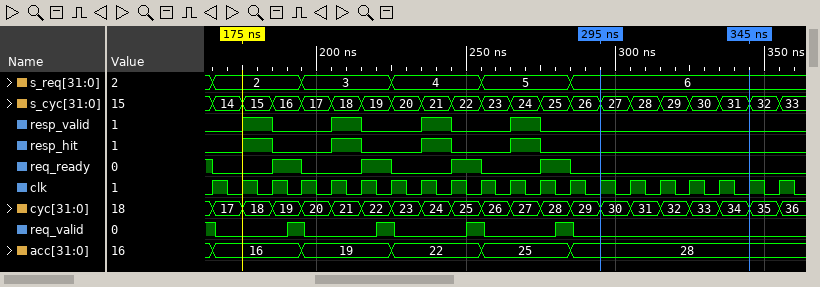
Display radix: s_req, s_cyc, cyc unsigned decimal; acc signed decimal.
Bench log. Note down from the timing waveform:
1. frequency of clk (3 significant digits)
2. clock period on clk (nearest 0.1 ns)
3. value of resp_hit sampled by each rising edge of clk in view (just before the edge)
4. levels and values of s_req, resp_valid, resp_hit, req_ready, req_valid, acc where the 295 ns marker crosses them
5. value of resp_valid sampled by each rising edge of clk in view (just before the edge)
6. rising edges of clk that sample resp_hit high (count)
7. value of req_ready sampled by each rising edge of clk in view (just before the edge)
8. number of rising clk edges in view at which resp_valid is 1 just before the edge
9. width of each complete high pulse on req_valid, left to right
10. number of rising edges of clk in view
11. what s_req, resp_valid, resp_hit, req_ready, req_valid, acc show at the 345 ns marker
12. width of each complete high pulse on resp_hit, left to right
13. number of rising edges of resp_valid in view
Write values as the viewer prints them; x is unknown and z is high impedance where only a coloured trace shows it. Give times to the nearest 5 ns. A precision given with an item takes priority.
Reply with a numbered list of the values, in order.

1. 100 MHz
2. 10 ns
3. 0 0 1 0 0 1 0 0 1 0 0 1 0 0 0 0 0 0 0 0
4. s_req=6, resp_valid=0, resp_hit=0, req_ready=0, req_valid=0, acc=28
5. 0 0 1 0 0 1 0 0 1 0 0 1 0 0 0 0 0 0 0 0
6. 4
7. 1 0 0 1 0 0 1 0 0 1 0 0 1 0 0 0 0 0 0 0
8. 4
9. 5 ns, 5 ns, 5 ns, 5 ns
10. 20
11. s_req=6, resp_valid=0, resp_hit=0, req_ready=0, req_valid=0, acc=28
12. 10 ns, 10 ns, 10 ns, 10 ns
13. 4
